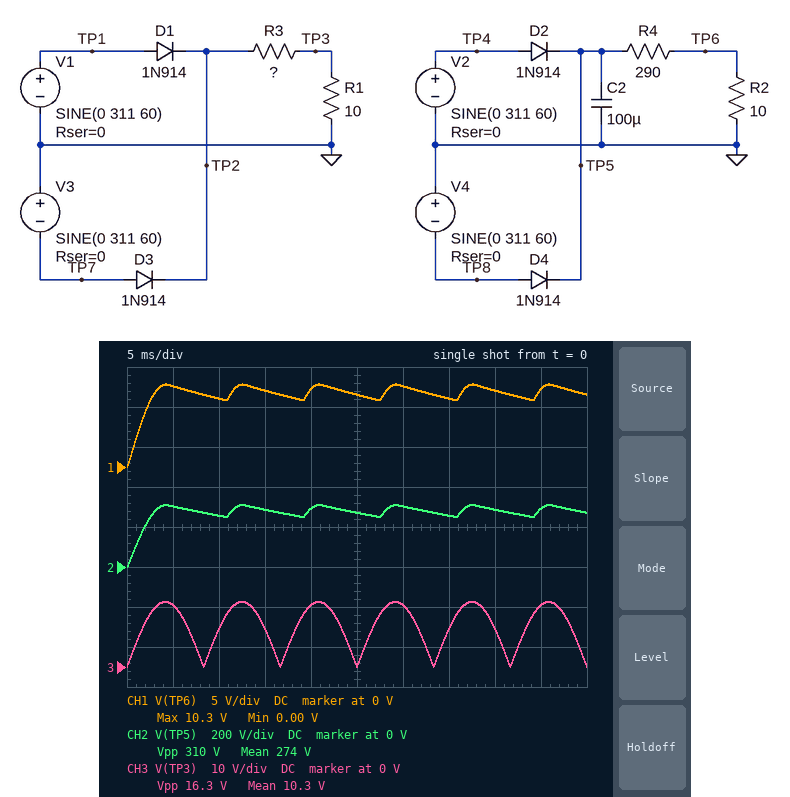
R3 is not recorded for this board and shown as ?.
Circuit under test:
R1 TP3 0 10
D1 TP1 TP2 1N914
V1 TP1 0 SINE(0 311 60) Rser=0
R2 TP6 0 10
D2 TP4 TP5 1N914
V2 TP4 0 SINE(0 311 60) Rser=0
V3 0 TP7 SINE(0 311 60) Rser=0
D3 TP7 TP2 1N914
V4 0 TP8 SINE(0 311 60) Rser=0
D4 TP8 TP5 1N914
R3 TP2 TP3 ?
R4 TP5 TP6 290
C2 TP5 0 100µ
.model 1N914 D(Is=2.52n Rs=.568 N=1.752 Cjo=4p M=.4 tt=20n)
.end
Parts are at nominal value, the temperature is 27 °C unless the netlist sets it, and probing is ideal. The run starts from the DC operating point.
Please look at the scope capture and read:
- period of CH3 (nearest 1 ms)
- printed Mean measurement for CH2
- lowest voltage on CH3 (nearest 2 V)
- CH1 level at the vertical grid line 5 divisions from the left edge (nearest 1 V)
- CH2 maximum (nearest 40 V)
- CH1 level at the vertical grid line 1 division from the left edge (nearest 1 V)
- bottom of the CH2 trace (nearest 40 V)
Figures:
8 ms
274 V
0 V
9 V
320 V
10 V
0 V
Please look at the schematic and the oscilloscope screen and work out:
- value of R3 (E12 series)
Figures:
180 Ω
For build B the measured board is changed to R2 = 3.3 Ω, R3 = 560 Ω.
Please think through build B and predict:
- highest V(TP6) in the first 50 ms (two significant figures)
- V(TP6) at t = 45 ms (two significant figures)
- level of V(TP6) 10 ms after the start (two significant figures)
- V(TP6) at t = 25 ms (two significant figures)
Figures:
3.5 V
3.3 V
2.9 V
3.0 V
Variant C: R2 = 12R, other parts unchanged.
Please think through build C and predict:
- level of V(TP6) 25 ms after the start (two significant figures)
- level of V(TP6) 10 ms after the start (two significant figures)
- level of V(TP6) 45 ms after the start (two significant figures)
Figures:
11 V
10 V
12 V
